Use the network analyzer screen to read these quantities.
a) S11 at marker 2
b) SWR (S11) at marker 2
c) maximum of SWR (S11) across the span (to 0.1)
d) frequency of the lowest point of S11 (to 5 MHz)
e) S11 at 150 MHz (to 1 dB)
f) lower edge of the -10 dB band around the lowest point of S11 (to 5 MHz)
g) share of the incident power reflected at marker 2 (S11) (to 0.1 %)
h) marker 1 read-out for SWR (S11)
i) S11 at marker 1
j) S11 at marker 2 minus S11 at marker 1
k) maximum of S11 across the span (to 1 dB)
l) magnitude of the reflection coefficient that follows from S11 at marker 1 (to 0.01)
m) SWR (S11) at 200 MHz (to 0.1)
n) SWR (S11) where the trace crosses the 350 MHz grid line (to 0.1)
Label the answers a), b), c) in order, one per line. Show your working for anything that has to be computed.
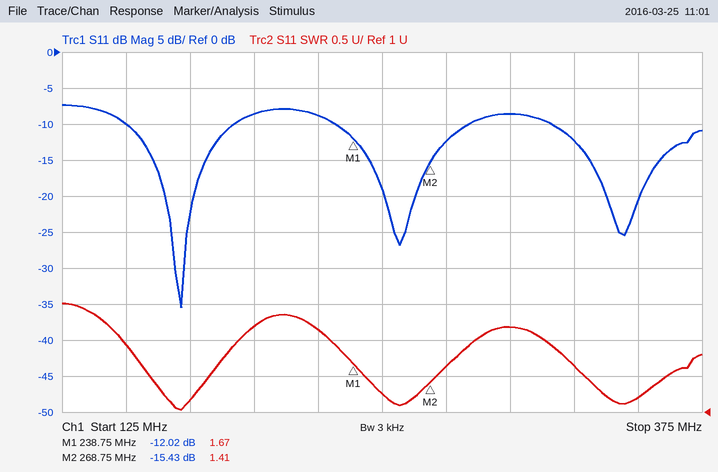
a) -15.43 dB
b) 1.41
c) 2.5
d) 170 MHz
e) -10 dB
f) 150 MHz
g) 10^(-15.43/10) ≈ 2.9 %
h) 1.67
i) -12.02 dB
j) -15.43 − (-12.02) = -3.41 dB
k) -7 dB
l) 10^(-12.02/20) ≈ 0.25
m) 2.2
n) 1.2
